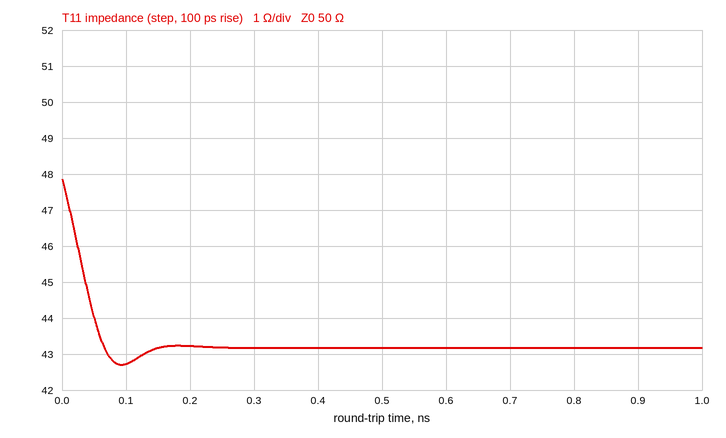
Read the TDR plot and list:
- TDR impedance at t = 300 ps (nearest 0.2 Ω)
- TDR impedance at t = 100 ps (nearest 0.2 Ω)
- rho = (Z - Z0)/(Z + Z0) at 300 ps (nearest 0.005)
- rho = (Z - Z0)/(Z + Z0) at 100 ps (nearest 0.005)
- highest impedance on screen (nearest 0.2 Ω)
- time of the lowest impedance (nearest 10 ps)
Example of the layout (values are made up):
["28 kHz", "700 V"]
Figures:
["43.2 Ω", "42.8 Ω", "-0.075", "-0.080", "47.8 Ω", "90 ps"]
